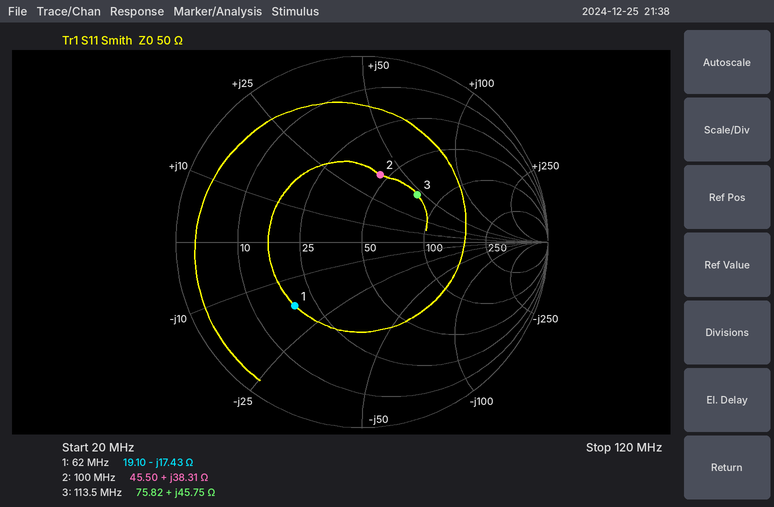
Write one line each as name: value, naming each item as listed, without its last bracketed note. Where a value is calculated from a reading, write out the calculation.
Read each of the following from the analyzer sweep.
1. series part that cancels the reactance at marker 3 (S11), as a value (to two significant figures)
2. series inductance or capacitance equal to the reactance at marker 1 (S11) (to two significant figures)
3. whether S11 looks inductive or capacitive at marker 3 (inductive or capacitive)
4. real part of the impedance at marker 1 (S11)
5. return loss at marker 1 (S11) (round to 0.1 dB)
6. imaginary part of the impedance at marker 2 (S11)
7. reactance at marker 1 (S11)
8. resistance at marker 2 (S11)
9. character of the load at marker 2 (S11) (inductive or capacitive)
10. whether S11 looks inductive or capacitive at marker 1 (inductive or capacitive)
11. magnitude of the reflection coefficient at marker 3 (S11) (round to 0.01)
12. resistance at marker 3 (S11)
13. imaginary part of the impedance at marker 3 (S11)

series part that cancels the reactance at marker 3 (S11), as a value: C = 1/(2π × 113.5 MHz × 45.75 Ω) ≈ 31 pF
series inductance or capacitance equal to the reactance at marker 1 (S11): C = 1/(2π × 62 MHz × 17.43 Ω) ≈ 147 pF, so 150 pF to two significant figures
whether S11 looks inductive or capacitive at marker 3: inductive
real part of the impedance at marker 1: 19.10 Ω
return loss at marker 1 (S11): 6.1 dB
imaginary part of the impedance at marker 2: +38.31 Ω
reactance at marker 1: -17.43 Ω
resistance at marker 2: 45.50 Ω
character of the load at marker 2 (S11): inductive
whether S11 looks inductive or capacitive at marker 1: capacitive
magnitude of the reflection coefficient at marker 3 (S11): 0.39
resistance at marker 3: 75.82 Ω
imaginary part of the impedance at marker 3: +45.75 Ω
